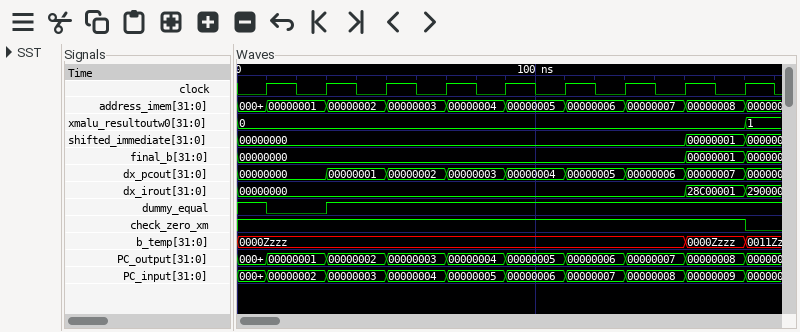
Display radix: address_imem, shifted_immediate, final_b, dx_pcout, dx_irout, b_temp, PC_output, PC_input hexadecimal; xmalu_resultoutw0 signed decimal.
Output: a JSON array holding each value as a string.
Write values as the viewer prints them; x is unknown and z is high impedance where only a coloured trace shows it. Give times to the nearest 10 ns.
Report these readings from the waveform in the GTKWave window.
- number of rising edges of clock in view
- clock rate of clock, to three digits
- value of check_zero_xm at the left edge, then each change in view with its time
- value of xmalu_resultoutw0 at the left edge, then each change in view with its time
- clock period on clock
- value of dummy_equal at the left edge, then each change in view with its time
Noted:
["9", "50.0 MHz", "1, 0 at 170 ns", "0, 1 at 170 ns", "20 ns", "1, 0 at 10 ns, 1 at 30 ns"]
